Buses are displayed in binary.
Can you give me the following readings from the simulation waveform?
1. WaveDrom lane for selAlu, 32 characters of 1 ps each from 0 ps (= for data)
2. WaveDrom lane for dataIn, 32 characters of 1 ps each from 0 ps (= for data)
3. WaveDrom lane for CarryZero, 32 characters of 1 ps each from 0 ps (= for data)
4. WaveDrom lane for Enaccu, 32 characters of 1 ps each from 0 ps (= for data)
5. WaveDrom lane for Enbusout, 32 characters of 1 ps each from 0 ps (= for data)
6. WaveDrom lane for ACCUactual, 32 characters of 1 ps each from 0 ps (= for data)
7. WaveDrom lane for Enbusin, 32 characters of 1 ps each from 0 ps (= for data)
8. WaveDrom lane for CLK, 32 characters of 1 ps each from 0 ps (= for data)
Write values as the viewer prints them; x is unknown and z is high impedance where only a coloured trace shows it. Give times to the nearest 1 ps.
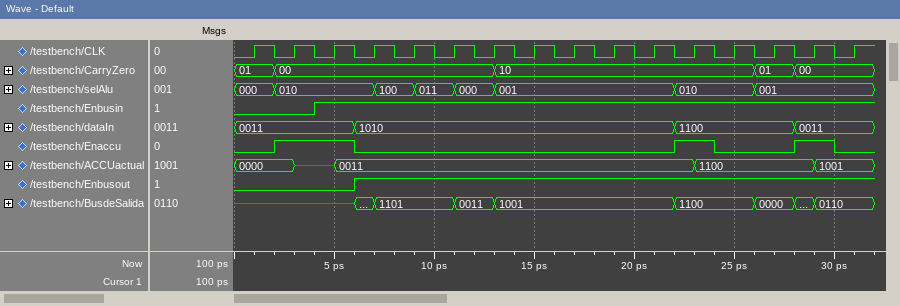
{name: 'selAlu', wave: '=.=....=.=.=.=........=...=.....', data: '000 010 100 011 000 001 010 001'}
{name: 'dataIn', wave: '=.....=...............=.....=...', data: '0011 1010 1100 0011'}
{name: 'CarryZero', wave: '=.=..........=............=.=...', data: '01 00 10 01 00'}
{name: 'Enaccu', wave: '0.1...0...............1.0...1.0.'}
{name: 'Enbusout', wave: '0.....1.........................'}
{name: 'ACCUactual', wave: '=..z.=.................=.....=..', data: '0000 0011 1100 1001'}
{name: 'Enbusin', wave: '0...1...........................'}
{name: 'CLK', wave: '01010101010101010101010101010101'}
